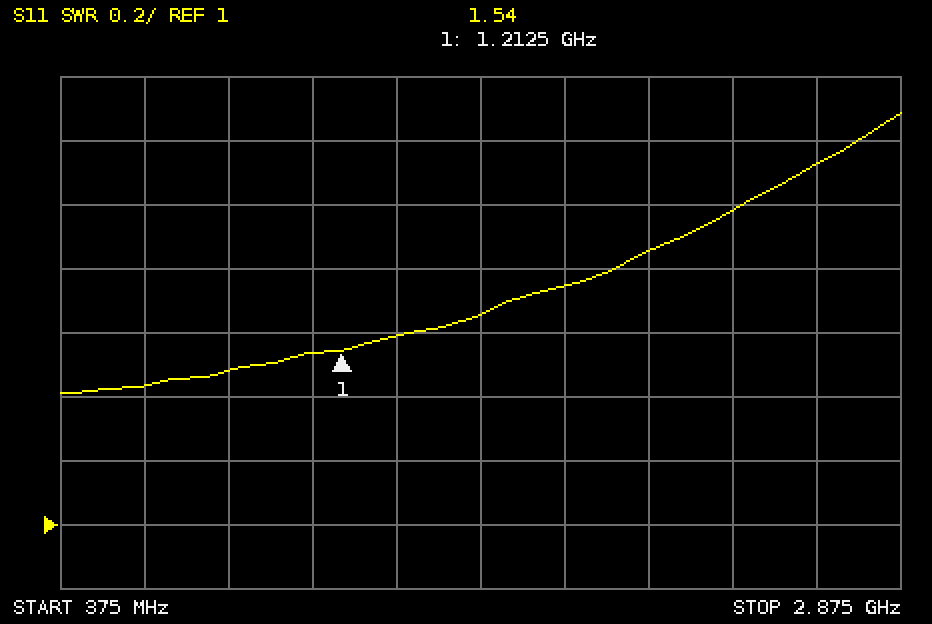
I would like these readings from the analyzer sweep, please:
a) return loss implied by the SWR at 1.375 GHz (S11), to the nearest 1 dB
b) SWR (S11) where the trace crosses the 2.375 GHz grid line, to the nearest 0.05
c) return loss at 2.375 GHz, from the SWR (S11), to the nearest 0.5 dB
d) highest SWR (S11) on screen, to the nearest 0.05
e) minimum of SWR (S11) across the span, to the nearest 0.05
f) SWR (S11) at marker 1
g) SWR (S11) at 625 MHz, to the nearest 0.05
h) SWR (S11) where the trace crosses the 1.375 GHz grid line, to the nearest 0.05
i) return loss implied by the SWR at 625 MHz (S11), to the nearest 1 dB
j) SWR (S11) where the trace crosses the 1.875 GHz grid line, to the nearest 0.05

13 dB
2.00
9.5 dB
2.30
1.40
1.54
1.45
1.60
15 dB
1.75
